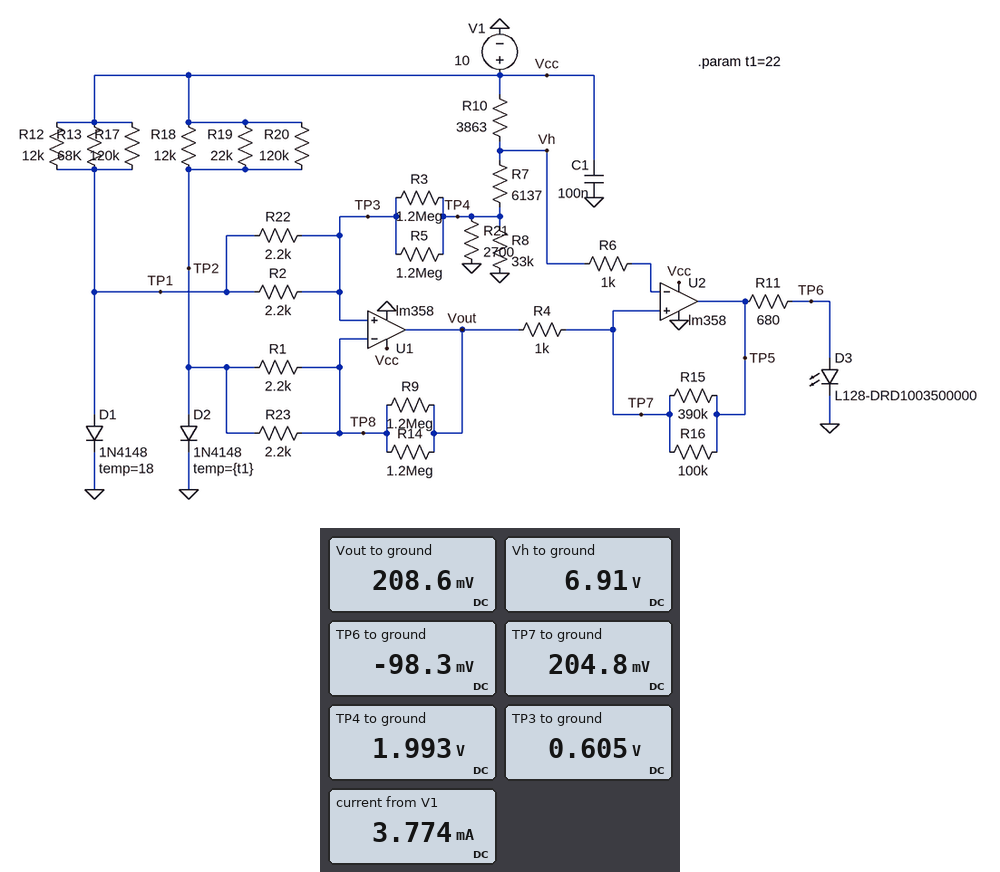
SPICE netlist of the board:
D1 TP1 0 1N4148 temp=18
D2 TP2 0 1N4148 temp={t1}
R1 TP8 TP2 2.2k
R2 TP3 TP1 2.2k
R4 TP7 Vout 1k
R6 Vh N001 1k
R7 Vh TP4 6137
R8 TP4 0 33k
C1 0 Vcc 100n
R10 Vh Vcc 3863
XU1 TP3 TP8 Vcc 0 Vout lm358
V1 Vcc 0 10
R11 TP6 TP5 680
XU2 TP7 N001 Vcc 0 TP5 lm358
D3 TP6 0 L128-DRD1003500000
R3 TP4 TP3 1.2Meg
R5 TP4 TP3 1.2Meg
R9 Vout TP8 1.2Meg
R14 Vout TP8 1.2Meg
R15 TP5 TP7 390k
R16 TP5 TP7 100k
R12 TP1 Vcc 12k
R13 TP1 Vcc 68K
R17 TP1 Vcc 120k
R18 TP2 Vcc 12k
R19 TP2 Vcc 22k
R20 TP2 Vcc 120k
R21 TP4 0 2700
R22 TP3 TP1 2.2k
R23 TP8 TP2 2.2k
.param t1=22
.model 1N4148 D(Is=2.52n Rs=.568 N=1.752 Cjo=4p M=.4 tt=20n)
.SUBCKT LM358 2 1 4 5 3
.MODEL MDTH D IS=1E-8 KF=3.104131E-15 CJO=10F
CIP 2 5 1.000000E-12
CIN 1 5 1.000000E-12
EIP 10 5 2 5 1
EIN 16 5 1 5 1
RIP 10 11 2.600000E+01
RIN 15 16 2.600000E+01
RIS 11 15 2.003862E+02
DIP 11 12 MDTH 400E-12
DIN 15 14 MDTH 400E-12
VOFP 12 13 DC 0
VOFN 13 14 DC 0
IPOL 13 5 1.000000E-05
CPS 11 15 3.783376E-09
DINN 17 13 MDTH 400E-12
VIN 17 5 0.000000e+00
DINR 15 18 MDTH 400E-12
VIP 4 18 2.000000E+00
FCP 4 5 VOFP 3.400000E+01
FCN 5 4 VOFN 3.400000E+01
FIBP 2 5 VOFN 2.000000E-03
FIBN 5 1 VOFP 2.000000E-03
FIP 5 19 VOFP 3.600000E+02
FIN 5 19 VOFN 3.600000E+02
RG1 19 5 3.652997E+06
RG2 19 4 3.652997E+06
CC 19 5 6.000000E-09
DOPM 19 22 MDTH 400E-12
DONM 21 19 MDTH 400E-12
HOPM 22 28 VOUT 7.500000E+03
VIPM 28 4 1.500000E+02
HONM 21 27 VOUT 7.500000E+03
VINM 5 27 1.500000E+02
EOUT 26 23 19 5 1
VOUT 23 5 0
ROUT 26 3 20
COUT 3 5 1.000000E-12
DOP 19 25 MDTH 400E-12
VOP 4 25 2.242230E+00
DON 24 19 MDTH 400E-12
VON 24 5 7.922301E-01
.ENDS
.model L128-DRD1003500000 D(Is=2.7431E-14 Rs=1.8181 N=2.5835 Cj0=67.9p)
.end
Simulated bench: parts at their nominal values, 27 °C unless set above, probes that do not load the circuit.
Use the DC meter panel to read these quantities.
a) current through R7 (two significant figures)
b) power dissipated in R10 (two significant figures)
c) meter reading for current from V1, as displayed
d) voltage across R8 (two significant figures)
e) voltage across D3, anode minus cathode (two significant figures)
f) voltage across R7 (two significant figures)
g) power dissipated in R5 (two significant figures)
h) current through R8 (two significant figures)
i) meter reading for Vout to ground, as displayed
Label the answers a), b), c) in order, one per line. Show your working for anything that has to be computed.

a) (6.91 V - 1.993 V) / 6.137 kΩ = 800 µA
b) (10 V - 6.91 V)^2 / 3.863 kΩ = 2.5 mW
c) 3.774 mA
d) 1.993 V = 2.0 V
e) -98.3 mV = -98 mV
f) 6.91 V - 1.993 V = 4.9 V
g) (1.993 V - 605 mV)^2 / 1.2 MΩ = 1.6 µW
h) (1.993 V) / 33 kΩ = 60 µA
i) 208.6 mV
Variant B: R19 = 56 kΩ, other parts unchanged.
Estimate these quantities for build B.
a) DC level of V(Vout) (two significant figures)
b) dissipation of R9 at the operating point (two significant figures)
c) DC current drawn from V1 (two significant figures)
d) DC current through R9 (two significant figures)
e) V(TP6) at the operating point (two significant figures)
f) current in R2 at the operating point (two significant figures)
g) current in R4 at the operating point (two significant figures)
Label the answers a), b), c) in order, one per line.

a) 5.5 V
b) 20 µW
c) 3.5 mA
d) 4.1 µA
e) -97 mV
f) 1.2 µA
g) 69 µA
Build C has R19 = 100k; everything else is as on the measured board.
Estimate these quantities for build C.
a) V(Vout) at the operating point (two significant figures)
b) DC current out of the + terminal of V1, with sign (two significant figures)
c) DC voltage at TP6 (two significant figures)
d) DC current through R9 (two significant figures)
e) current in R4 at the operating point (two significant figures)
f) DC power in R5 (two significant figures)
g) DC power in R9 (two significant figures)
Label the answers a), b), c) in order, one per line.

a) 7.2 V
b) -160 µA
c) 1.8 V
d) 5.5 µA
e) 15 µA
f) 1.6 µW
g) 36 µW
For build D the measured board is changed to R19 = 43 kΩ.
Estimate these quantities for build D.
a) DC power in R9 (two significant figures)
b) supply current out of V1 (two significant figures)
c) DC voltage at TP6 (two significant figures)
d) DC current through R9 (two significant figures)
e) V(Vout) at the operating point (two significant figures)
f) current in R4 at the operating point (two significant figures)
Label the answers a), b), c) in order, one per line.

a) 12 µW
b) 3.6 mA
c) -97 mV
d) 3.1 µA
e) 4.4 V
f) 55 µA
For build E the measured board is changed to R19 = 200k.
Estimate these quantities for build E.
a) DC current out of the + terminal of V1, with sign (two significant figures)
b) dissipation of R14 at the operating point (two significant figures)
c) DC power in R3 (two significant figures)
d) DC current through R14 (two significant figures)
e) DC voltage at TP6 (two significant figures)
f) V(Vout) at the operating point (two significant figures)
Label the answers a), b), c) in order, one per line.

a) -210 µA
b) 50 µW
c) 1.6 µW
d) 6.5 µA
e) 1.8 V
f) 8.4 V
